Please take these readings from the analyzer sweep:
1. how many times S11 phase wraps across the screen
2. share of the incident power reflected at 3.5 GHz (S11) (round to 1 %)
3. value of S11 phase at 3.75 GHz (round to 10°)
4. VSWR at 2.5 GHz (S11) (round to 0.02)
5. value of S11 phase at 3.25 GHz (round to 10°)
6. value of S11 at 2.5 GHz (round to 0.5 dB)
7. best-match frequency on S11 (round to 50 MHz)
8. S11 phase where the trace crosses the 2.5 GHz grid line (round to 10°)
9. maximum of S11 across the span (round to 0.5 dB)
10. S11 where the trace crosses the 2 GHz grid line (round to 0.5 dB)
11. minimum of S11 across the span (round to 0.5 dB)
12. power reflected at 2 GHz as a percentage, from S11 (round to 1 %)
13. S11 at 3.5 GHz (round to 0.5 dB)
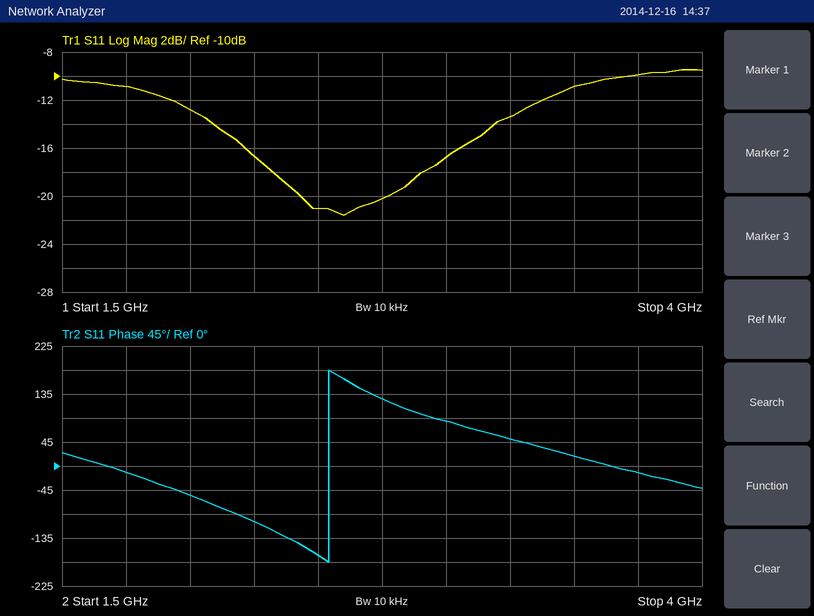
1
8 %
-10°
1.20
50°
-21.0 dB
2.60 GHz
-170°
-9.5 dB
-13.0 dB
-21.5 dB
5 %
-11.0 dB
